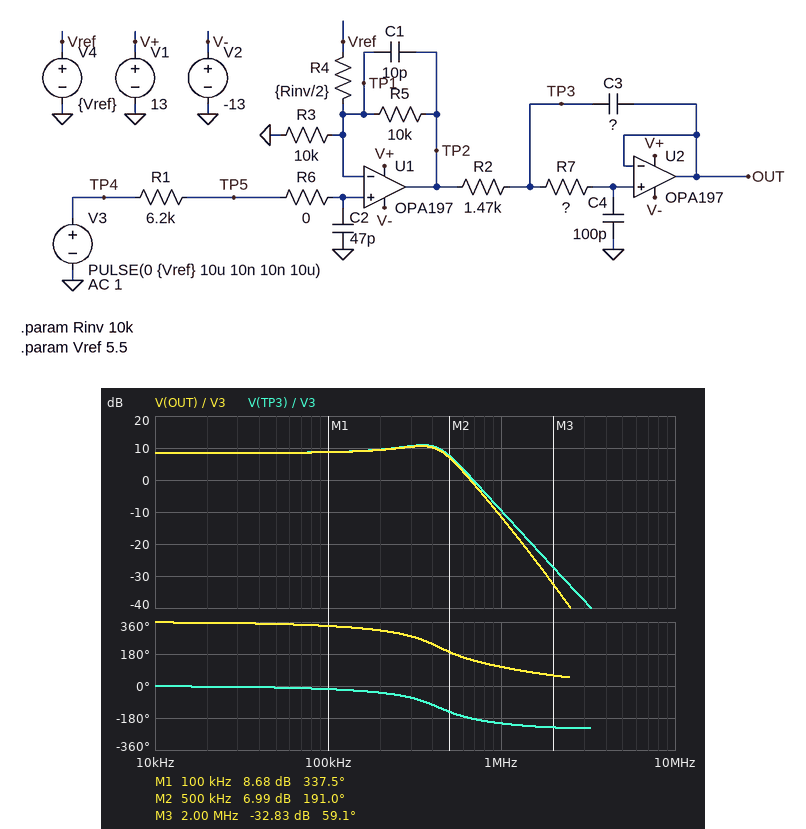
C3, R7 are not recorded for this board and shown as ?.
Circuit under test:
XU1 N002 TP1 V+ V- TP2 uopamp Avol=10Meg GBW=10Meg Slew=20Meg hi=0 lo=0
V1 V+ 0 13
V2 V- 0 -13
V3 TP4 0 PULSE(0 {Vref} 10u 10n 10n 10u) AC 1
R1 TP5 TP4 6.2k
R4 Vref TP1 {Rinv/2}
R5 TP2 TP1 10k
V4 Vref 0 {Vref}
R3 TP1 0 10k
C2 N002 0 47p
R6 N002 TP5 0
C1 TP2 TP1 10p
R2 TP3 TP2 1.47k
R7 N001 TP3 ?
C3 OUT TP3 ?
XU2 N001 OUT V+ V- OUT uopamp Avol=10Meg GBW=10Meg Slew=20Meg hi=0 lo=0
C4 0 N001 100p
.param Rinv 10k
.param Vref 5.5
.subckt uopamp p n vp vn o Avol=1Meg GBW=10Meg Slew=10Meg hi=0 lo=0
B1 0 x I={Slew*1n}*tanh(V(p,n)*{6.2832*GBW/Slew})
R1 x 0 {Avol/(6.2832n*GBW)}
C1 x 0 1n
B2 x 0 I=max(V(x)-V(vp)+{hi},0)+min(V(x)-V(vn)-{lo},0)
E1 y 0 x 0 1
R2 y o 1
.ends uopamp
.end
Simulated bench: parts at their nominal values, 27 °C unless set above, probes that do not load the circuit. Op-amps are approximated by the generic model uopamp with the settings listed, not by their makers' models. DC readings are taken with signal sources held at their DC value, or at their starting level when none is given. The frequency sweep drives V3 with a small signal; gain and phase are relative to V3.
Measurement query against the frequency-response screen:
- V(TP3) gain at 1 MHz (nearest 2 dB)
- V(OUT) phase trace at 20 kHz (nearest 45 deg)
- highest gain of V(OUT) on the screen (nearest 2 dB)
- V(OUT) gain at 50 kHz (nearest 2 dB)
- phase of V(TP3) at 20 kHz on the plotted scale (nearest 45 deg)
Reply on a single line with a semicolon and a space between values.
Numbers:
-10 dB; 360 deg; 10 dB; 8 dB; 0 deg
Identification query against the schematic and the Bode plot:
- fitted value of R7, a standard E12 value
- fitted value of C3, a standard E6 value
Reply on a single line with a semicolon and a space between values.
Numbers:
1.2 kΩ; 680 pF
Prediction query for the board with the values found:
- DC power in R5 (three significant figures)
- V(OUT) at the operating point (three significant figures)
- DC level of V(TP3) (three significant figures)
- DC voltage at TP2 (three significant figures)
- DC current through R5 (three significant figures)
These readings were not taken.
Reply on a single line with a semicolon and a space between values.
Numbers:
12.1 mW; -11.0 V; -11.0 V; -11.0 V; 1.10 mA
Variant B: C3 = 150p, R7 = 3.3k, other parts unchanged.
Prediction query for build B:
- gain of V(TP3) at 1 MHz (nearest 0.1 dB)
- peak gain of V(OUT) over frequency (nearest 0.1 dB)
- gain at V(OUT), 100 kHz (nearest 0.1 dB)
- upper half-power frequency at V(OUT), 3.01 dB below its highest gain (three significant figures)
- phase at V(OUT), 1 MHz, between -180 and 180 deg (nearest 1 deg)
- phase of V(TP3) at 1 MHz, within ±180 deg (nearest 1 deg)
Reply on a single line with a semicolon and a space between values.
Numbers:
-2.2 dB; 8.4 dB; 8.2 dB; 354 kHz; 141 deg; -149 deg
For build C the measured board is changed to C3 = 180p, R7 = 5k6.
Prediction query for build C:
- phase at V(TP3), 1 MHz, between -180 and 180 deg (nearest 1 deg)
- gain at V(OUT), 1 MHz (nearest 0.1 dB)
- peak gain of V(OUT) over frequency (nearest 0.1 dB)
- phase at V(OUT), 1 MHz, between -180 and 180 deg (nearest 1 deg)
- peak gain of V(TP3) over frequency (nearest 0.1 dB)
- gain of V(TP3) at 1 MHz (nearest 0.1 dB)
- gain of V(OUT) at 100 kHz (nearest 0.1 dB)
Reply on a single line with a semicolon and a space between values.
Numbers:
-153 deg; -14.8 dB; 8.4 dB; 127 deg; 8.5 dB; -3.5 dB; 8.0 dB
